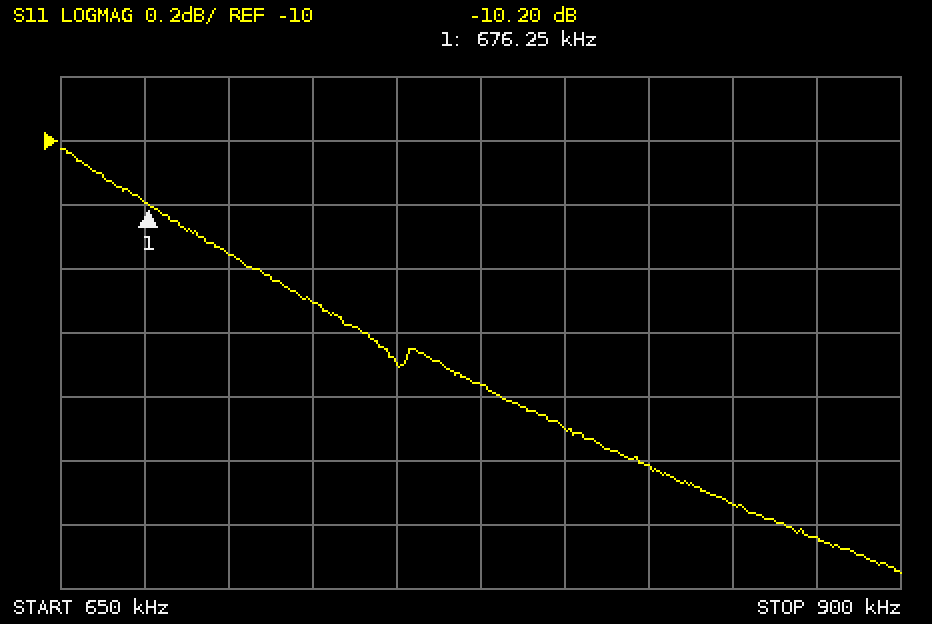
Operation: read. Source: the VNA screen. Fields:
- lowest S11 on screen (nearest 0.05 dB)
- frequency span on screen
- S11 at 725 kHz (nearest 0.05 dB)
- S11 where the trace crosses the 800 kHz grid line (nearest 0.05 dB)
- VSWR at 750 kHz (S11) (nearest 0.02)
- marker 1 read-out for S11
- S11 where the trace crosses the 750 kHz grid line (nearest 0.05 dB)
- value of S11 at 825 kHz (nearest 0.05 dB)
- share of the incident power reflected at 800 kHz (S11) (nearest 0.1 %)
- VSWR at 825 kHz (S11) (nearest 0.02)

-11.35 dB
250 kHz
-10.50 dB
-10.90 dB
1.82
-10.20 dB
-10.70 dB
-11.00 dB
8.1 %
1.78
